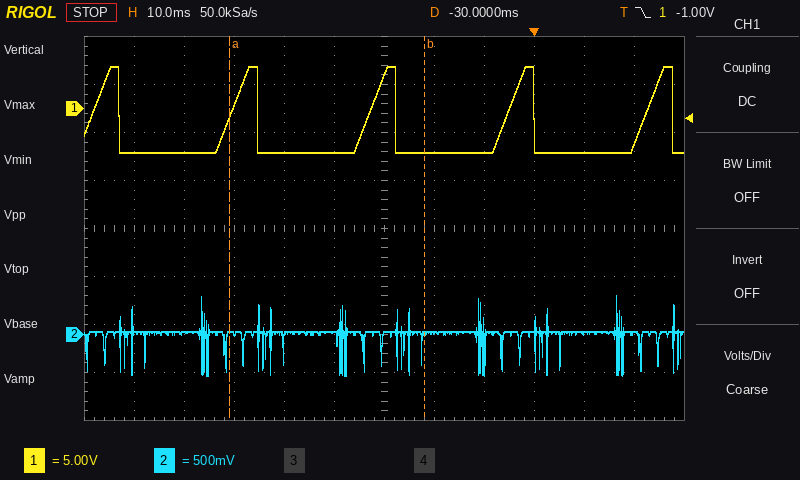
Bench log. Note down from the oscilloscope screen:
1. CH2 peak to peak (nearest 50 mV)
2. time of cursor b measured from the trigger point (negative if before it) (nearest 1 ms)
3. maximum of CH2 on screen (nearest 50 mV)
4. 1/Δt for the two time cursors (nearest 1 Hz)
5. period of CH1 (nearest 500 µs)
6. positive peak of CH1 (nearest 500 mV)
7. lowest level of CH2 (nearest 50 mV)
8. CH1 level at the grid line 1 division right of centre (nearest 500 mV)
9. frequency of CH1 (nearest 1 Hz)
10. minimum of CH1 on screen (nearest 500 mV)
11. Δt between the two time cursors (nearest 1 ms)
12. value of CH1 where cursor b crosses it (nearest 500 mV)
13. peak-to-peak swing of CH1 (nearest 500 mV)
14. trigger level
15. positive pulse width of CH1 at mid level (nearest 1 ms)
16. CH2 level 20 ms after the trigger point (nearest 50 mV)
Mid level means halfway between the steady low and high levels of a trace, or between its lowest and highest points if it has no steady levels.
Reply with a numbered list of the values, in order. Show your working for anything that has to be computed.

1. 400 mV − (-450 mV) = 850 mV
2. -22 ms
3. 400 mV
4. 1 / 39 ms ≈ 26 Hz
5. 27.5 ms
6. 4.5 V
7. -450 mV
8. -4.5 V
9. 1 / 27.5 ms ≈ 36 Hz
10. -4.5 V
11. 39 ms
12. -4.5 V
13. 4.5 V − (-4.5 V) = 9.0 V
14. -1.00 V
15. 5 ms
16. 0 mV
